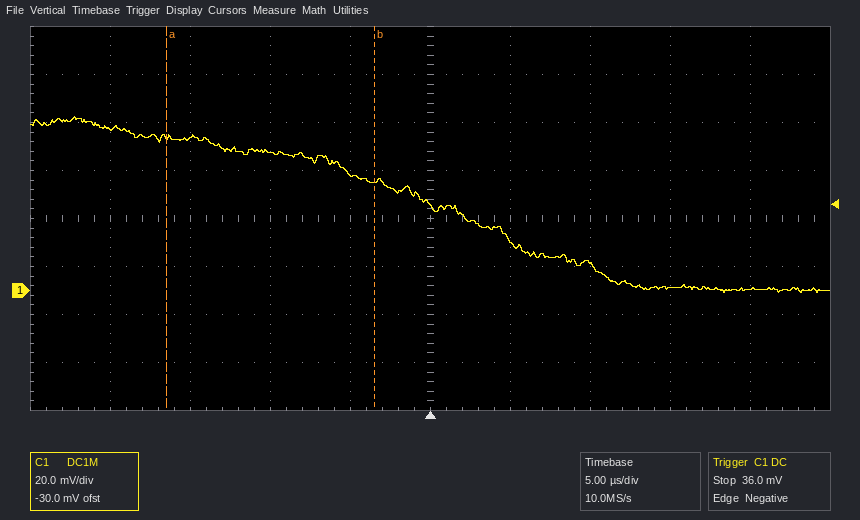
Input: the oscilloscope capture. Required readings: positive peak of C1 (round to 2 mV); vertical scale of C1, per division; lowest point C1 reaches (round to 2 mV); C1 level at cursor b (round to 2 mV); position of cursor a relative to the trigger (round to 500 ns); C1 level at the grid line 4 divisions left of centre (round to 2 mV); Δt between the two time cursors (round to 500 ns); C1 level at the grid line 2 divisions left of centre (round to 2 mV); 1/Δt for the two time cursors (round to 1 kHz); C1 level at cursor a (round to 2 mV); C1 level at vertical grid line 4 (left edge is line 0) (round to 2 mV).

72 mV
20 mV
0 mV
46 mV
-16.5 µs
68 mV
13.0 µs
58 mV
77 kHz
64 mV
48 mV
